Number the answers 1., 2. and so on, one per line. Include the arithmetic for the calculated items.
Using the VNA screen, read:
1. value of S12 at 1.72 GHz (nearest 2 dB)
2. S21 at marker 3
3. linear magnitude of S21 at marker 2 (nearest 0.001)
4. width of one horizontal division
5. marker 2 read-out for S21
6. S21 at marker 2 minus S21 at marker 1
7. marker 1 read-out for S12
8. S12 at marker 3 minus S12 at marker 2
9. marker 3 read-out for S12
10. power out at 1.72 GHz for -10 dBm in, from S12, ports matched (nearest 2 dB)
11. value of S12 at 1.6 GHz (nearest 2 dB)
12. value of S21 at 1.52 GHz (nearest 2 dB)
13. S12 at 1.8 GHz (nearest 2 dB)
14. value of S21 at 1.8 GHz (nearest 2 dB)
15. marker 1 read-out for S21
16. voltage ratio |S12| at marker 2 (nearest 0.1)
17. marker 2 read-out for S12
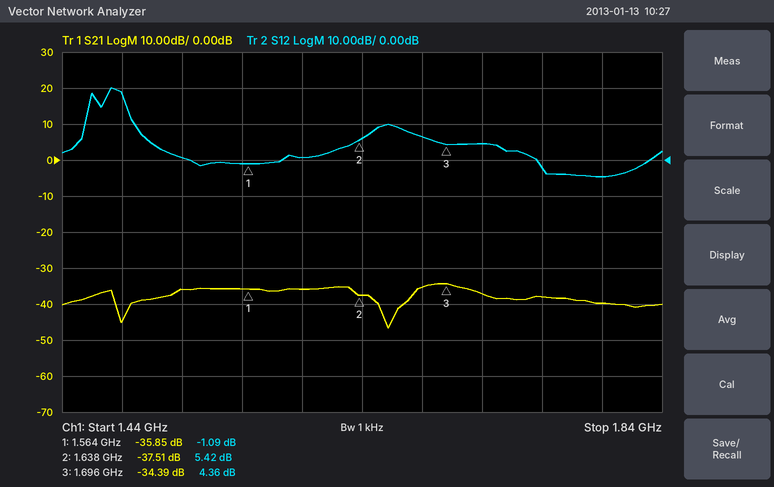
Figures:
1. 4 dB
2. -34.39 dB
3. 10^(-37.51/20) ≈ 0.013
4. 40 MHz
5. -37.51 dB
6. -37.51 − (-35.85) = -1.66 dB
7. -1.09 dB
8. 4.36 − (5.42) = -1.06 dB
9. 4.36 dB
10. -10 dBm + (4 dB) = -6 dBm
11. 0 dB
12. -36 dB
13. -4 dB
14. -40 dB
15. -35.85 dB
16. 10^(5.42/20) ≈ 1.9
17. 5.42 dB
